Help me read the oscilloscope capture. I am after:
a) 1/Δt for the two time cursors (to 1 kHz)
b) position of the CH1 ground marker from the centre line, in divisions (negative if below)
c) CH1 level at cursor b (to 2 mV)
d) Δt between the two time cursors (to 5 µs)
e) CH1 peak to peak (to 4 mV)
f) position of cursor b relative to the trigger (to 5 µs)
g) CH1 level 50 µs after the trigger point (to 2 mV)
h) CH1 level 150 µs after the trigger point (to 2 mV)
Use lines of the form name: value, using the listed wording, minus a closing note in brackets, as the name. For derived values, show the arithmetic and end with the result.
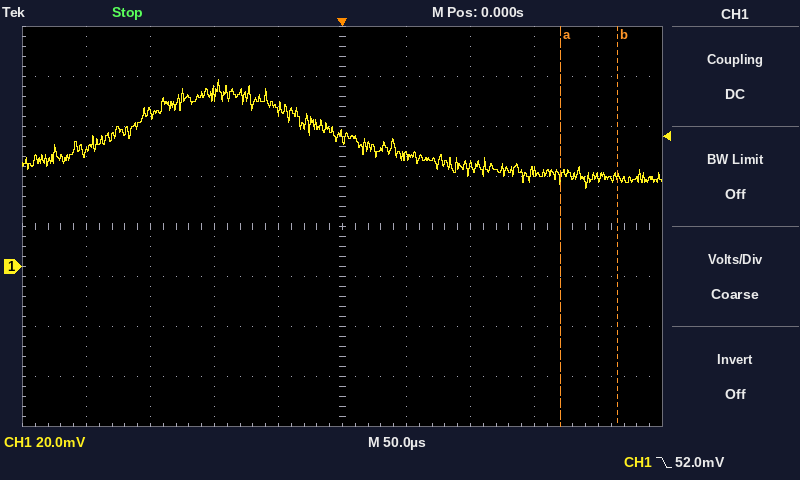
1/Δt for the two time cursors: 1 / 45 µs ≈ 22 kHz
position of the CH1 ground marker from the centre line, in divisions: -0.8 div
CH1 level at cursor b: 36 mV
Δt between the two time cursors: 45 µs
CH1 peak to peak: 44 mV
position of cursor b relative to the trigger: +215 µs
CH1 level 50 µs after the trigger point: 44 mV
CH1 level 150 µs after the trigger point: 38 mV
